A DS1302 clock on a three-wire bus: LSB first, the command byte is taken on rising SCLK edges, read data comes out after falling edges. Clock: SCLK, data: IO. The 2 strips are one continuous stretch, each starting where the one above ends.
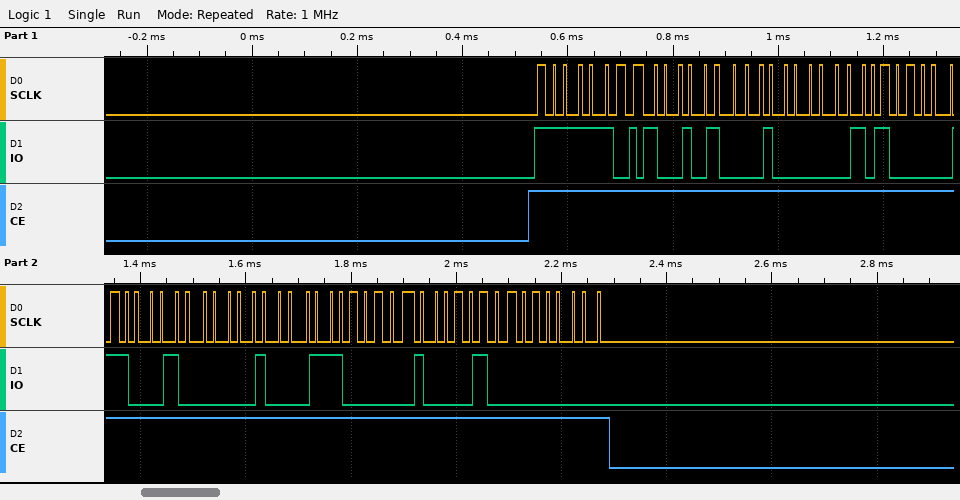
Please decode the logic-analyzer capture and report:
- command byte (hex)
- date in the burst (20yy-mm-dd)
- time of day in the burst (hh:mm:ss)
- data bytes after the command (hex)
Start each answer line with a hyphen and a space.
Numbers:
- 0xBF
- 2021-10-23
- 05:02:29
- 29 02 05 23 10 07 21 00
